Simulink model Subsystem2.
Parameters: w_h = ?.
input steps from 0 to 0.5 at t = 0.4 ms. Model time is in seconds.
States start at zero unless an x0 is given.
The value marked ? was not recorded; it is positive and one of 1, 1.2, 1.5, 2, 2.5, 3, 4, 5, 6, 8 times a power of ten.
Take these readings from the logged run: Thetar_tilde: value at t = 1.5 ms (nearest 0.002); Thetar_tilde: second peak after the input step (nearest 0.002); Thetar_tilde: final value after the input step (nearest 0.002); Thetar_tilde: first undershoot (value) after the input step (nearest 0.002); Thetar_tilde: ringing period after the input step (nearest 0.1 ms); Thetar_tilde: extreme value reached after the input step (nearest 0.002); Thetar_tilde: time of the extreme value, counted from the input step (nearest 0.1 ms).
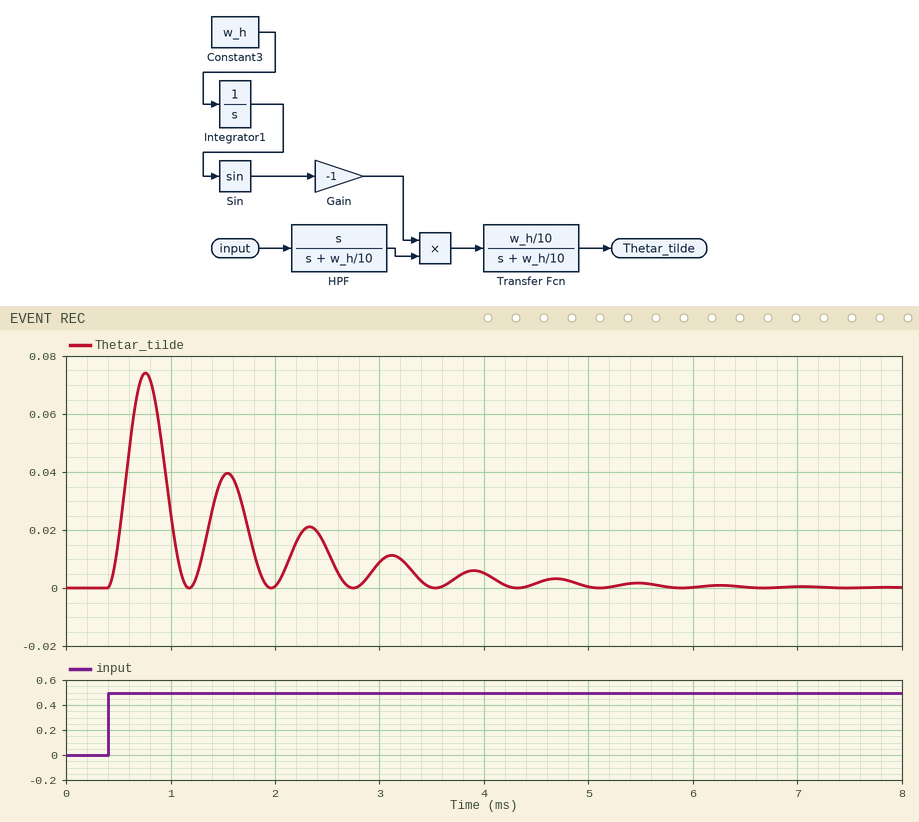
0.038
0.040
0.000
0.000
0.8 ms
0.074
0.4 ms
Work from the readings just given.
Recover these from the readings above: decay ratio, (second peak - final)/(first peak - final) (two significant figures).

0.54
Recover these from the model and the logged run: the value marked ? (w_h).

8000
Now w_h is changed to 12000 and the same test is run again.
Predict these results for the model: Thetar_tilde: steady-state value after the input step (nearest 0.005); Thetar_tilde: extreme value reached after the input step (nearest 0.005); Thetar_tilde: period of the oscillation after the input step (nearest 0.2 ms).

0.000
0.040
0.6 ms
